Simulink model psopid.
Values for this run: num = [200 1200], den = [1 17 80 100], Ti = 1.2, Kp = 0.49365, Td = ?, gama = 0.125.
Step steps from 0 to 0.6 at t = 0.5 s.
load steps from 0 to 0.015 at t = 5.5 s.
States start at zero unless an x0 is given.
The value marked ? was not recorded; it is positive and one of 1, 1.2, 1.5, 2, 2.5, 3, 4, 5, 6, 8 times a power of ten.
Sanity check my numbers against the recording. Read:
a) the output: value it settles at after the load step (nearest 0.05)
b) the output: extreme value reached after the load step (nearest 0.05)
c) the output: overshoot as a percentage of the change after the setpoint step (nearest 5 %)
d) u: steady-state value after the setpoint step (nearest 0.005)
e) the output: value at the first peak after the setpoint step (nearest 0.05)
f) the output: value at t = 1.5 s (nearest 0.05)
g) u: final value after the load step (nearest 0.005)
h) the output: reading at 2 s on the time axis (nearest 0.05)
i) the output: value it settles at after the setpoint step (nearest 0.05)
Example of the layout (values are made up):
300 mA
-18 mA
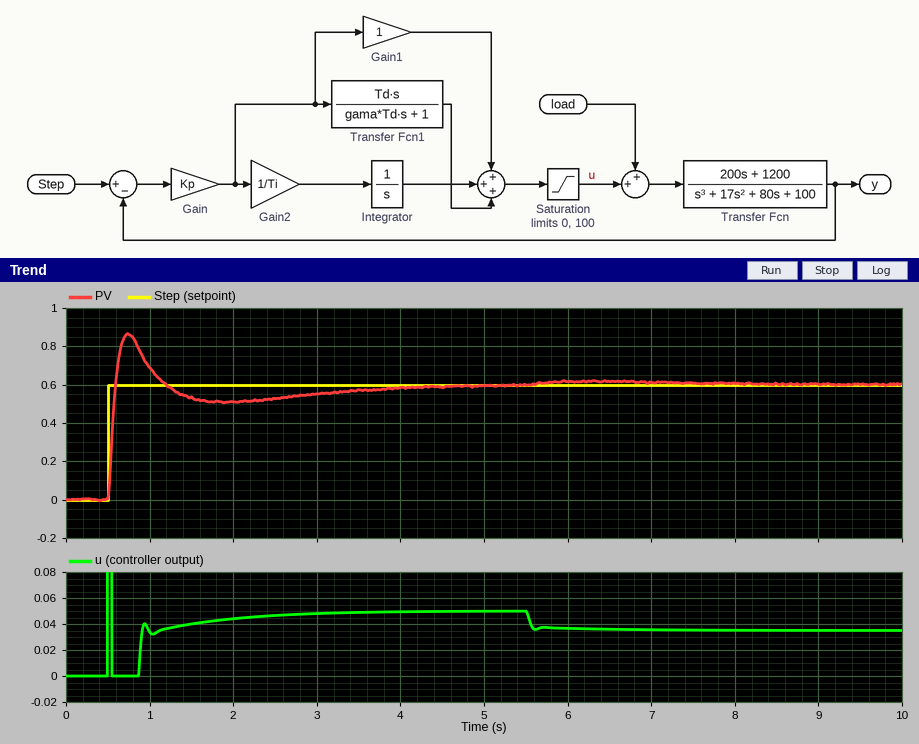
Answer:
0.60
0.60
45 %
0.050
0.85
0.55
0.035
0.50
0.60
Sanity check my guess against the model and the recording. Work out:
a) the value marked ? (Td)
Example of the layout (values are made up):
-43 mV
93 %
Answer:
0.3
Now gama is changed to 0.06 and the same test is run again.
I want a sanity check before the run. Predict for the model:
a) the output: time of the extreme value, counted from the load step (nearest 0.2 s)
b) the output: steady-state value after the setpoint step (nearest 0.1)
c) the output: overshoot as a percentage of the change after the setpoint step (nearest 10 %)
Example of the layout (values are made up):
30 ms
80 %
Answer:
0.8 s
0.6
60 %
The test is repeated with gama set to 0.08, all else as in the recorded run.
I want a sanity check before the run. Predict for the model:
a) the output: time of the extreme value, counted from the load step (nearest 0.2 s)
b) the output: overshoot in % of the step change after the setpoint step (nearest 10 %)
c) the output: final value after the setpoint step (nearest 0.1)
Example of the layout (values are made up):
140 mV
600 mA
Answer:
0.8 s
50 %
0.6
